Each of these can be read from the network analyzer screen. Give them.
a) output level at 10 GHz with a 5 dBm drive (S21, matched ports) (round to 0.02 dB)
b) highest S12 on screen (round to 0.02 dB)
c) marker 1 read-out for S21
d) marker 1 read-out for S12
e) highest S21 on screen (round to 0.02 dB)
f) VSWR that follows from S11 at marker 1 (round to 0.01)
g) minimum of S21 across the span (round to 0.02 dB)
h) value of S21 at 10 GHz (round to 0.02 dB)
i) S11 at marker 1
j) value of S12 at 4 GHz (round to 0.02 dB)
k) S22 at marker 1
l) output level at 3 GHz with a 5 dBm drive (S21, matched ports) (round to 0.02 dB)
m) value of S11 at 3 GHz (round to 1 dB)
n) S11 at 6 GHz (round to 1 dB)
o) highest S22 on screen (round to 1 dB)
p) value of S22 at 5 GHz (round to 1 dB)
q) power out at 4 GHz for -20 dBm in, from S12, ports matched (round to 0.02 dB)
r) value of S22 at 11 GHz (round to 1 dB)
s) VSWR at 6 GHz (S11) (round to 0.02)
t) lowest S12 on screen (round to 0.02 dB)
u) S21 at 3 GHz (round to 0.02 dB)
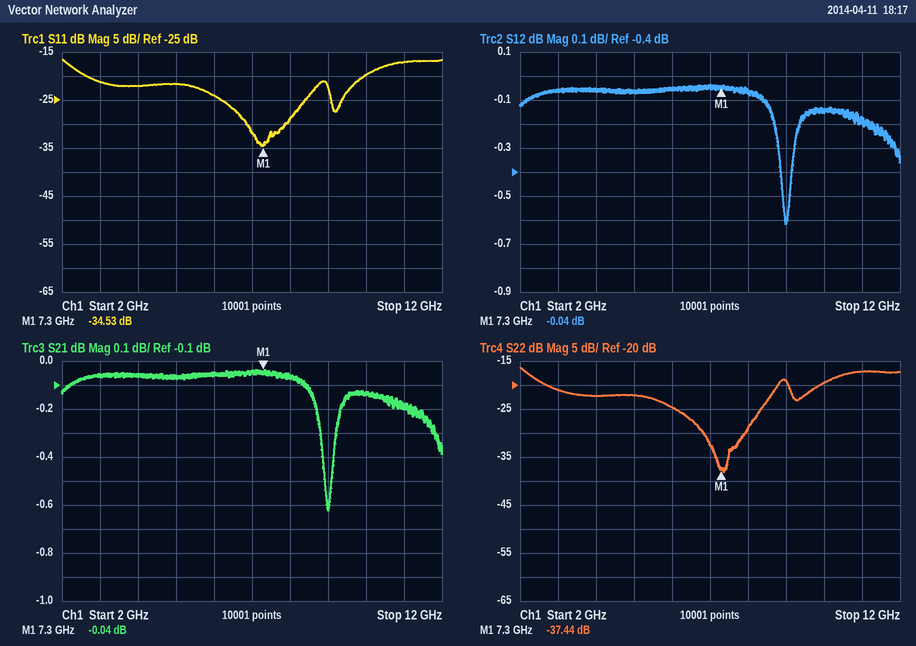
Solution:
4.86 dBm
-0.04 dB
-0.04 dB
-0.04 dB
-0.04 dB
1.04
-0.62 dB
-0.14 dB
-34.53 dB
-0.06 dB
-37.44 dB
4.94 dBm
-21 dB
-24 dB
-16 dB
-22 dB
-20.06 dBm
-17 dB
1.14
-0.62 dB
-0.06 dB
